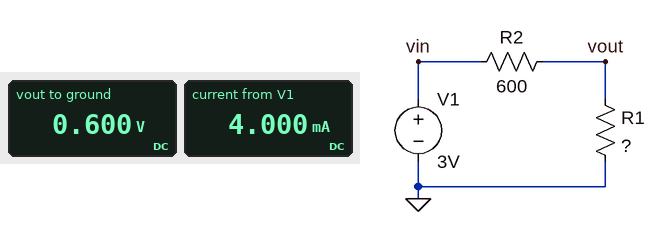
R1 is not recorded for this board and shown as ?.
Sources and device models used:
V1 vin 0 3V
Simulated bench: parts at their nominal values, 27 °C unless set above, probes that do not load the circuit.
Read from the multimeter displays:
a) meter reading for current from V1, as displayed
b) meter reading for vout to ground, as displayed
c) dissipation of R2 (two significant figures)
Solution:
4.000 mA
0.600 V
9.6 mW
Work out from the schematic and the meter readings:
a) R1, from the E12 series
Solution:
150 Ω
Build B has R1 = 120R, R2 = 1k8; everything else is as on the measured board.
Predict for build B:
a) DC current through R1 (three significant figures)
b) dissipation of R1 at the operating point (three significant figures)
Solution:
1.56 mA
293 µW
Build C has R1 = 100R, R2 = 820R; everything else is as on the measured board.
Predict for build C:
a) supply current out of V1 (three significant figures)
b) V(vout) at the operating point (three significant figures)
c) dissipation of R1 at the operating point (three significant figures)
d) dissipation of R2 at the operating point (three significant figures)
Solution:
3.26 mA
326 mV
1.06 mW
8.72 mW
